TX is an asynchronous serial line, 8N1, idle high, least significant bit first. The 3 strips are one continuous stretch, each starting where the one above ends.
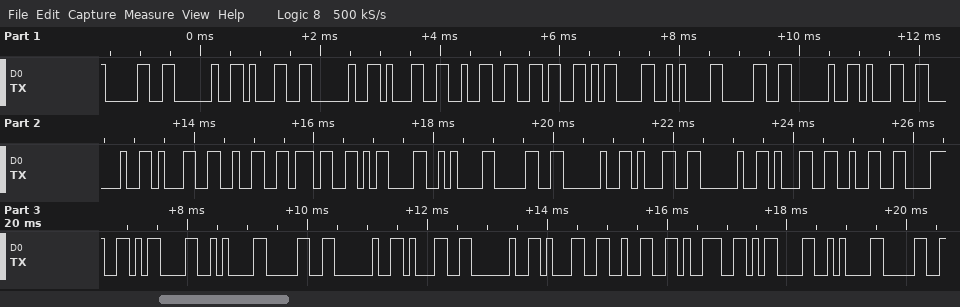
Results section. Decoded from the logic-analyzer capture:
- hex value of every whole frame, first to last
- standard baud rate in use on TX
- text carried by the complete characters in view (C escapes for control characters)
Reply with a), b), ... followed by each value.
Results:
a) 30 20 31 20 31 32 36 0D 0A 30 20 31 20 31 32 37 0D 0A 30 20 31 20 31 32 38 0D 0A 30 20 31 20 31 32 39 0D 0A 30
b) 9600 baud
c) "0 1 126\r\n0 1 127\r\n0 1 128\r\n0 1 129\r\n0"
